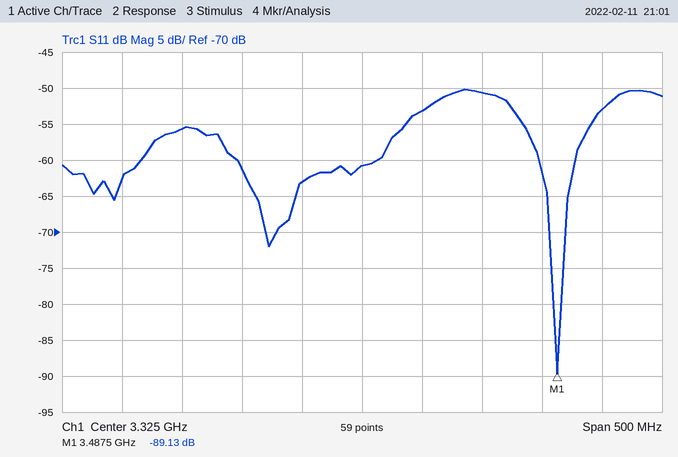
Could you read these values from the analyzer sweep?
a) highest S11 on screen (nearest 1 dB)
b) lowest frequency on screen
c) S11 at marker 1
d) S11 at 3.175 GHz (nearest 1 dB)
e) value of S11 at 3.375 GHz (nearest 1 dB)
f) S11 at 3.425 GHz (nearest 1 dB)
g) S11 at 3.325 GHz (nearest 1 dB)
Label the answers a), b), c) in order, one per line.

a) -50 dB
b) 3.075 GHz
c) -89.13 dB
d) -56 dB
e) -53 dB
f) -51 dB
g) -61 dB
